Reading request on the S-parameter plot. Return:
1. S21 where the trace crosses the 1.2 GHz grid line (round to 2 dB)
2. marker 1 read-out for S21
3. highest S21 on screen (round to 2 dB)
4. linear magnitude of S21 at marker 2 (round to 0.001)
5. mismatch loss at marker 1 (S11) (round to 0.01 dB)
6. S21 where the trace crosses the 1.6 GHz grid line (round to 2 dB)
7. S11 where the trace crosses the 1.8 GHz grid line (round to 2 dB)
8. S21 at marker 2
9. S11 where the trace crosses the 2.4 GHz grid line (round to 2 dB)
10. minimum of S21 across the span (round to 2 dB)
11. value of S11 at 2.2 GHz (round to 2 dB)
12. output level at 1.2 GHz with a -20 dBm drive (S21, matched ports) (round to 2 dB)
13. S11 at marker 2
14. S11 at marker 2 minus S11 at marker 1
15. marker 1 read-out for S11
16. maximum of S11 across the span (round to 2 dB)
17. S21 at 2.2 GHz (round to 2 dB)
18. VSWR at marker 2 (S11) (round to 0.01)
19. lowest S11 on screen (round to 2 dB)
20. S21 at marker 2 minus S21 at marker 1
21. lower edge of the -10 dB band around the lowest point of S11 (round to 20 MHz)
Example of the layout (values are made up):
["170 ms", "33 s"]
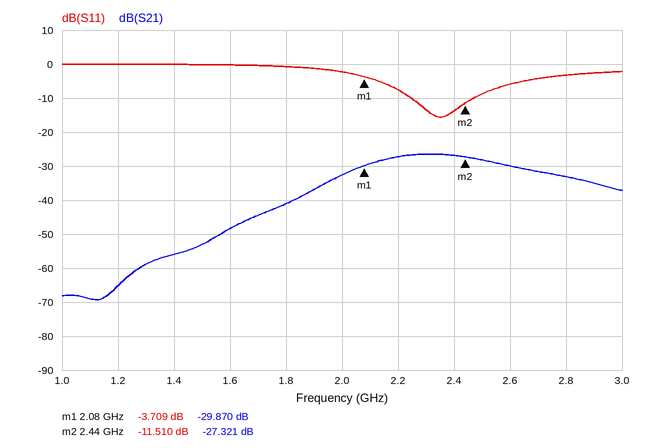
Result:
["-66 dB", "-29.870 dB", "-26 dB", "0.043", "2.41 dB", "-48 dB", "0 dB", "-27.321 dB", "-14 dB", "-70 dB", "-8 dB", "-86 dBm", "-11.510 dB", "-7.801 dB", "-3.709 dB", "0 dB", "-28 dB", "1.72", "-16 dB", "2.549 dB", "2.24 GHz"]
